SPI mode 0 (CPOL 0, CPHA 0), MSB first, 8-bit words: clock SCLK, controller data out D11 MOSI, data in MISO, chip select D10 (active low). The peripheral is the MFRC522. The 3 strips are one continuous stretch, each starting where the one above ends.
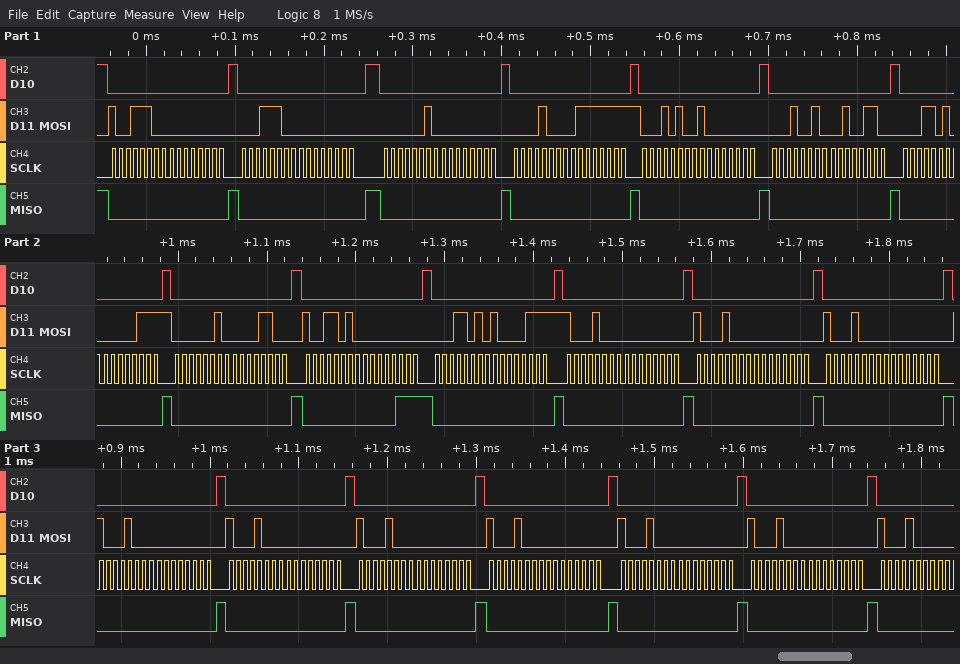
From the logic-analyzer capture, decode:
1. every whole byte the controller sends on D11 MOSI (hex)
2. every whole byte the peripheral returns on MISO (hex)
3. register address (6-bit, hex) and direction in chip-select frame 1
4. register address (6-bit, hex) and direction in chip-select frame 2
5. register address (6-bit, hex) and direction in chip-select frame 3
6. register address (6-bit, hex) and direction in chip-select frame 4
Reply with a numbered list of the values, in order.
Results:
1. 9C 00 1C 00 02 00 08 7F 14 80 12 26 1A 07 02 0C 9A 00 1A 87 88 00 88 00 88 00 88 00 88 00 88 00 88 00 88 00 88 00 88
2. 00 00 00 00 00 00 00 00 00 00 00 00 00 00 00 00 00 07 00 00 00 00 00 00 00 00 00 00 00 00 00 00 00 00 00 00 00 00 00
3. 0x0E read
4. 0x0E write
5. 0x01 write
6. 0x04 write
